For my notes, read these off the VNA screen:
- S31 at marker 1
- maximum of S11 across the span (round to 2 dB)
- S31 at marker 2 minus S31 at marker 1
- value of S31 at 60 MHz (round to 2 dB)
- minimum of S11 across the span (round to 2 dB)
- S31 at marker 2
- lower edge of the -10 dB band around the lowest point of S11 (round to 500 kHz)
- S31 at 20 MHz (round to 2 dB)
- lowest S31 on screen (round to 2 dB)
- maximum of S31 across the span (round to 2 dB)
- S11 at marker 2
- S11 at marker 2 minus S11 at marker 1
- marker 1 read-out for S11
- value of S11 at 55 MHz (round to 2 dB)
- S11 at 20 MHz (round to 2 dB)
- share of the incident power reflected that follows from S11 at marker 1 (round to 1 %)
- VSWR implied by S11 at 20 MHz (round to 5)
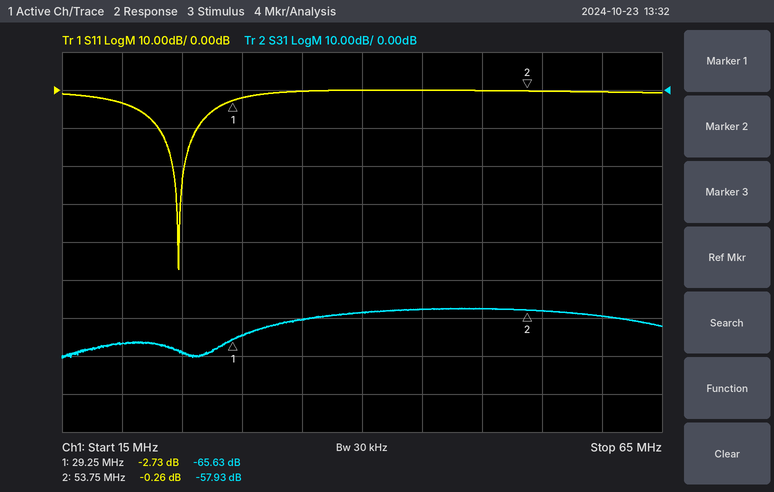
-65.63 dB
0 dB
7.70 dB
-60 dB
-48 dB
-57.93 dB
23.0 MHz
-66 dB
-70 dB
-58 dB
-0.26 dB
2.47 dB
-2.73 dB
0 dB
-4 dB
53 %
5
